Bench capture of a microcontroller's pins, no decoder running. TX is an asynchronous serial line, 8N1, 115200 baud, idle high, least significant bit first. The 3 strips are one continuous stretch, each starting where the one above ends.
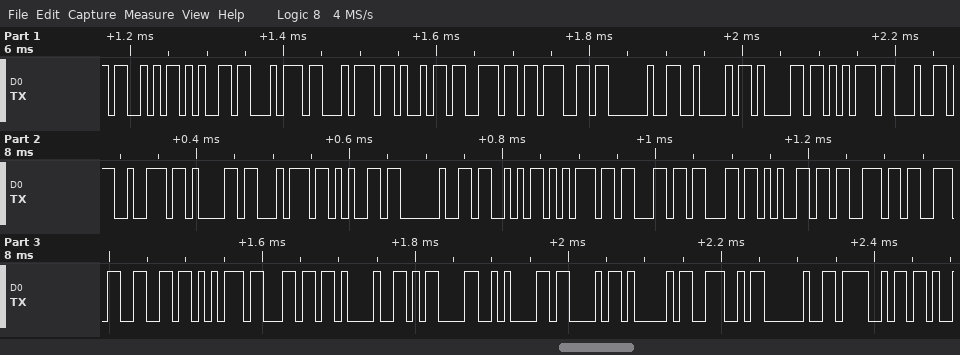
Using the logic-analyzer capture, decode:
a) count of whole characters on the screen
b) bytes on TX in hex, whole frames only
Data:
35
53 65 74 74 69 6E 67 20 42 61 75 64 72 61 74 65 20 53 75 63 63 65 73 73 66 75 6C 21 0D 0A 43 41 4E 20 4F
